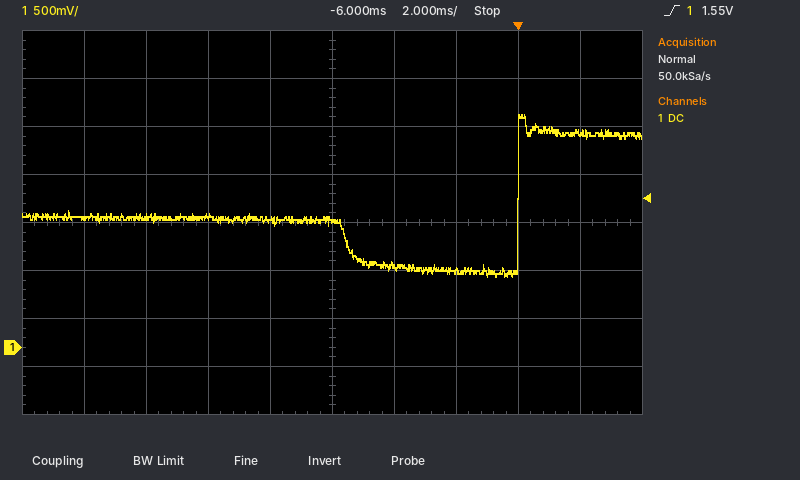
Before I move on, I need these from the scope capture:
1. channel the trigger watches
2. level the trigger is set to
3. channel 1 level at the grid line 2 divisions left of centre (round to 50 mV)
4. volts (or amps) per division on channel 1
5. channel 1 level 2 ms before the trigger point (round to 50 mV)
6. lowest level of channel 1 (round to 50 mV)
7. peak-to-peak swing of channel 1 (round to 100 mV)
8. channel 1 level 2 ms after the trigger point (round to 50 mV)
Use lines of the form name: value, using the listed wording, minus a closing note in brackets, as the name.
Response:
channel the trigger watches: channel 1
level the trigger is set to: 1.55 V
channel 1 level at the grid line 2 divisions left of centre: 1.35 V
volts (or amps) per division on channel 1: 500 mV
channel 1 level 2 ms before the trigger point: 800 mV
lowest level of channel 1: 750 mV
peak-to-peak swing of channel 1: 1.70 V
channel 1 level 2 ms after the trigger point: 2.25 V
